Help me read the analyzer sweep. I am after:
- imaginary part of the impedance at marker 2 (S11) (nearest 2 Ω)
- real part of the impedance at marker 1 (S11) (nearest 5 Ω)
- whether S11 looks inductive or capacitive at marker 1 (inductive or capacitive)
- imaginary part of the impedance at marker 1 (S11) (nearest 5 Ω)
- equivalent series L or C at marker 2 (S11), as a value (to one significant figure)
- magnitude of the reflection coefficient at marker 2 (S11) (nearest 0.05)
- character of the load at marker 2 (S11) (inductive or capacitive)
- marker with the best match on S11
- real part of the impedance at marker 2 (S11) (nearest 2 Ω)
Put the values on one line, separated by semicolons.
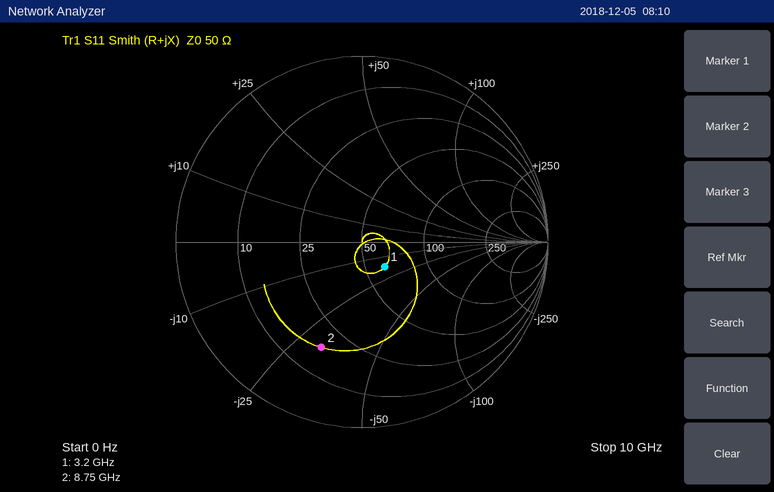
-32 Ω; 60 Ω; capacitive; -15 Ω; 600 fF; 0.60; capacitive; marker 1; 18 Ω
